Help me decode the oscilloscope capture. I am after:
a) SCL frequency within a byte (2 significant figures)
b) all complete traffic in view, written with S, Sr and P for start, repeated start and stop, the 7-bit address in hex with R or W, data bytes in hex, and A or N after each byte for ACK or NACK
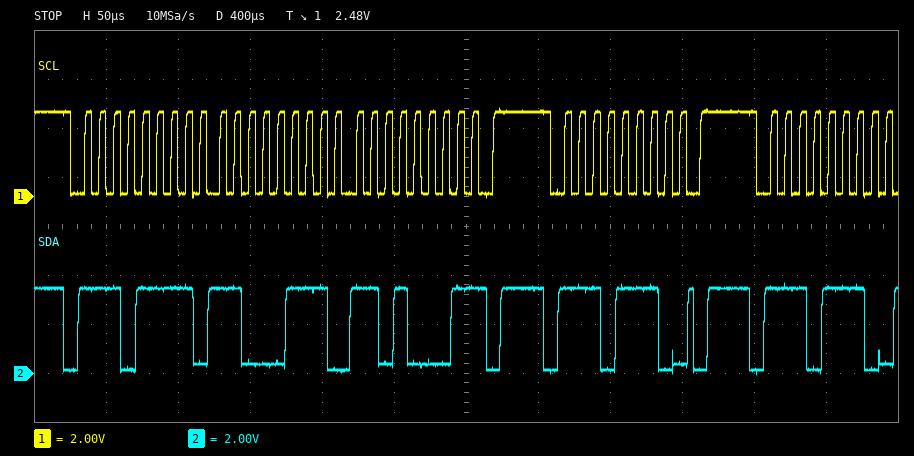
100 kHz
S 77R A C7 A D1 N P S 77W A P S 77W A
